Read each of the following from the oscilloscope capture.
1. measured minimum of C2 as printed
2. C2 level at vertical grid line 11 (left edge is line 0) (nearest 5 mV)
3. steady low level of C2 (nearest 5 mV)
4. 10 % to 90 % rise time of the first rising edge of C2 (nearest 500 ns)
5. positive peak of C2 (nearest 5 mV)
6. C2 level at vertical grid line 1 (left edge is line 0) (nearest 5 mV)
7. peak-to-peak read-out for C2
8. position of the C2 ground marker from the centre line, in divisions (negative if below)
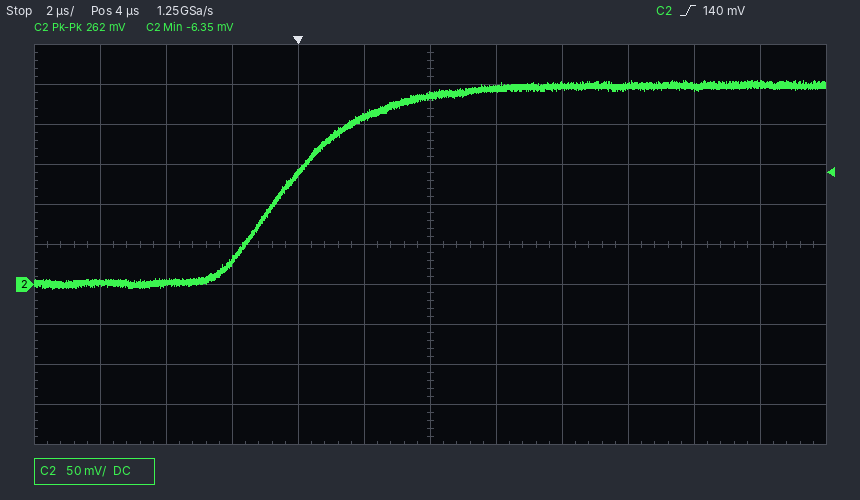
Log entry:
-6.35 mV
250 mV
0 mV
5.0 µs
255 mV
0 mV
262 mV
-1.0 div
